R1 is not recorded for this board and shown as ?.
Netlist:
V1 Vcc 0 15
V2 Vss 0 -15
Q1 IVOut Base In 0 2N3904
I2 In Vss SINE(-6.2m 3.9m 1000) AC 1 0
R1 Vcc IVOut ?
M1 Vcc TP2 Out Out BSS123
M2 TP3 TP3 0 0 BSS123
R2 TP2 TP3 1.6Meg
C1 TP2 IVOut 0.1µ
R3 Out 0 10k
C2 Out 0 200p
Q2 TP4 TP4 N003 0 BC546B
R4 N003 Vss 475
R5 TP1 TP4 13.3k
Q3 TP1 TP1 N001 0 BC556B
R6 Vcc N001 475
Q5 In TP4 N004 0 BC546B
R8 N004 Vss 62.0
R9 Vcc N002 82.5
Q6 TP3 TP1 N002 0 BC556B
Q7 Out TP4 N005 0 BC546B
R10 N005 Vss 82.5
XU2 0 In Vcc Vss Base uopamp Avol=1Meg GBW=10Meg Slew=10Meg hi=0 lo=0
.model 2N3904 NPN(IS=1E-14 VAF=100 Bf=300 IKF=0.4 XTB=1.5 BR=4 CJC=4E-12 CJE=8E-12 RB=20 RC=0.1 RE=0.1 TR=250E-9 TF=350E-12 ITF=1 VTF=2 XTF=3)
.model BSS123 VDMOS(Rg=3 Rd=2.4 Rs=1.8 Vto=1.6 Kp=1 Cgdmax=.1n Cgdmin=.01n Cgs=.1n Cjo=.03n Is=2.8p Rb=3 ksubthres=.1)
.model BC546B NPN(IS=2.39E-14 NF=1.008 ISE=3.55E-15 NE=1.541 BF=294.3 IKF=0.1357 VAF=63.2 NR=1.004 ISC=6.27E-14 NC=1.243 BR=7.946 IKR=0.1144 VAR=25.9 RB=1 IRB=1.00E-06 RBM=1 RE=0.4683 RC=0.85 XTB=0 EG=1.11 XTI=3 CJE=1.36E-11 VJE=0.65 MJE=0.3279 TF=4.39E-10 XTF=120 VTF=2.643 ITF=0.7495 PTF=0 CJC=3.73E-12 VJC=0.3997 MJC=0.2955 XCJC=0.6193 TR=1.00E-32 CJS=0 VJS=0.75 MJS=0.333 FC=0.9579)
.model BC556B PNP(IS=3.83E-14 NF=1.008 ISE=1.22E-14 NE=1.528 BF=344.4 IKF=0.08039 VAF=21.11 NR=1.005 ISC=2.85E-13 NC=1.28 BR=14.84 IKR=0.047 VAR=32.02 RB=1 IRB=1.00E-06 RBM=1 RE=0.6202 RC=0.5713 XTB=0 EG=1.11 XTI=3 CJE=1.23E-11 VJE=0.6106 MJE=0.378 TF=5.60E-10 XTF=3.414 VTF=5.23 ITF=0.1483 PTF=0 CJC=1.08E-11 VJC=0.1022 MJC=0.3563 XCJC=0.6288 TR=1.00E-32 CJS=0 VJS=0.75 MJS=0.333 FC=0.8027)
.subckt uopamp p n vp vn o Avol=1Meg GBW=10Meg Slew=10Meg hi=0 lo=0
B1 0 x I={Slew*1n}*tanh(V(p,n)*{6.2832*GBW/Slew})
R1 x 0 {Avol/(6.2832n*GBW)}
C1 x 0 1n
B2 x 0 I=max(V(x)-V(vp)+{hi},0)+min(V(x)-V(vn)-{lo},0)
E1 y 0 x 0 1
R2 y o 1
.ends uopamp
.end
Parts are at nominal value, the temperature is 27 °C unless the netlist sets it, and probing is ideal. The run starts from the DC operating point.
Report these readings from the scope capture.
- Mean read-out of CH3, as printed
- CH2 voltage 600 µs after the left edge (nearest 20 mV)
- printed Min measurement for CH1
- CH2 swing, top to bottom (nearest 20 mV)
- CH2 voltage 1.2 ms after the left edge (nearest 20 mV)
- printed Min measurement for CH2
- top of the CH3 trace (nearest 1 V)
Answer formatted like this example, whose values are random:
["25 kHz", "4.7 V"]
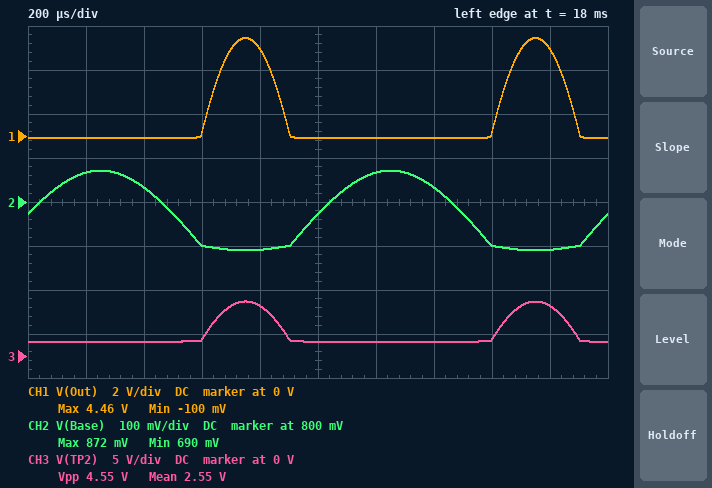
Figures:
["2.55 V", "700 mV", "-100 mV", "180 mV", "860 mV", "690 mV", "6 V"]
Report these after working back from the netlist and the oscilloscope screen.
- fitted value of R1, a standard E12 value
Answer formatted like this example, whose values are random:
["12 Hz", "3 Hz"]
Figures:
["2.7 kΩ"]
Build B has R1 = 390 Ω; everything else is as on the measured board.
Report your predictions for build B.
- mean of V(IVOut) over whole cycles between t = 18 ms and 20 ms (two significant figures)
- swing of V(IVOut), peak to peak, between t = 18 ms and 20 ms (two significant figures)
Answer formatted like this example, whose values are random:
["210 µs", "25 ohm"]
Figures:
["12 V", "3.0 V"]
